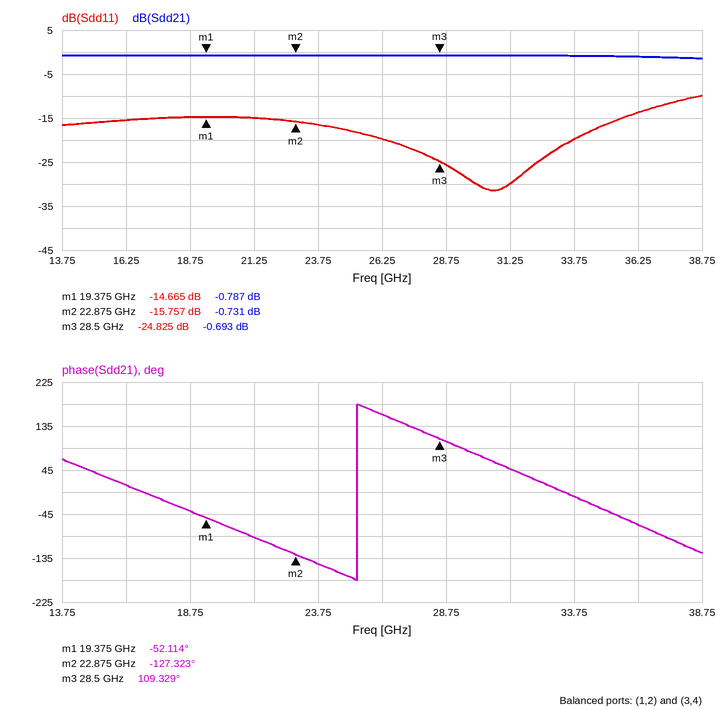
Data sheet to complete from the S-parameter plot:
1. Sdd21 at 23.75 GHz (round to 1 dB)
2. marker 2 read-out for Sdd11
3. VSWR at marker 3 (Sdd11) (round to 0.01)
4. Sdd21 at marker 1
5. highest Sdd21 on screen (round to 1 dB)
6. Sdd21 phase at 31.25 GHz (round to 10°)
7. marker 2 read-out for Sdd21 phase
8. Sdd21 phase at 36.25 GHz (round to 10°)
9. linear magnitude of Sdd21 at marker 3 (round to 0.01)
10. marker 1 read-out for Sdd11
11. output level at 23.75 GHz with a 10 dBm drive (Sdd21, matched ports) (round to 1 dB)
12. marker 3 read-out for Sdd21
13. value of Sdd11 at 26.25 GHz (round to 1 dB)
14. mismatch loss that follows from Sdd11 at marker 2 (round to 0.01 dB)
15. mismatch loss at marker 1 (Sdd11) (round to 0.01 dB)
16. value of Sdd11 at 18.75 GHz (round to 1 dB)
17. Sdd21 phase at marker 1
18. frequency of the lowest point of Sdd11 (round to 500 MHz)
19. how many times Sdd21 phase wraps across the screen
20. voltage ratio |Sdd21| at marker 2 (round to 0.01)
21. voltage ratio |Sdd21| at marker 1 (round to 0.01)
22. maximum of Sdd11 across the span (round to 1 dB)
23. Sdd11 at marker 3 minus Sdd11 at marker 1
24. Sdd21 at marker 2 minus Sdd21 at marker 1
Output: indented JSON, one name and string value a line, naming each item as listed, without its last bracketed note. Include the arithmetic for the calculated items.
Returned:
{
  "Sdd21 at 23.75 GHz": "-1 dB",
  "marker 2 read-out for Sdd11": "-15.757 dB",
  "VSWR at marker 3 (Sdd11)": "(1 + 0.0574)/(1 − 0.0574) ≈ 1.12",
  "Sdd21 at marker 1": "-0.787 dB",
  "highest Sdd21 on screen": "-1 dB",
  "Sdd21 phase at 31.25 GHz": "50°",
  "marker 2 read-out for Sdd21 phase": "-127.323°",
  "Sdd21 phase at 36.25 GHz": "-70°",
  "linear magnitude of Sdd21 at marker 3": "10^(-0.693/20) ≈ 0.92",
  "marker 1 read-out for Sdd11": "-14.665 dB",
  "output level at 23.75 GHz with a 10 dBm drive (Sdd21, matched ports)": "10 dBm + (-1 dB) = 9 dBm",
  "marker 3 read-out for Sdd21": "-0.693 dB",
  "value of Sdd11 at 26.25 GHz": "-20 dB",
  "mismatch loss that follows from Sdd11 at marker 2": "−10 log10(1 − 10^(-15.757/10)) ≈ 0.12 dB",
  "mismatch loss at marker 1 (Sdd11)": "−10 log10(1 − 10^(-14.665/10)) ≈ 0.15 dB",
  "value of Sdd11 at 18.75 GHz": "-15 dB",
  "Sdd21 phase at marker 1": "-52.114°",
  "frequency of the lowest point of Sdd11": "30.5 GHz",
  "how many times Sdd21 phase wraps across the screen": "1",
  "voltage ratio |Sdd21| at marker 2": "10^(-0.731/20) ≈ 0.92",
  "voltage ratio |Sdd21| at marker 1": "10^(-0.787/20) ≈ 0.91",
  "maximum of Sdd11 across the span": "-10 dB",
  "Sdd11 at marker 3 minus Sdd11 at marker 1": "-24.825 − (-14.665) = -10.160 dB",
  "Sdd21 at marker 2 minus Sdd21 at marker 1": "-0.731 − (-0.787) = 0.056 dB"
}
